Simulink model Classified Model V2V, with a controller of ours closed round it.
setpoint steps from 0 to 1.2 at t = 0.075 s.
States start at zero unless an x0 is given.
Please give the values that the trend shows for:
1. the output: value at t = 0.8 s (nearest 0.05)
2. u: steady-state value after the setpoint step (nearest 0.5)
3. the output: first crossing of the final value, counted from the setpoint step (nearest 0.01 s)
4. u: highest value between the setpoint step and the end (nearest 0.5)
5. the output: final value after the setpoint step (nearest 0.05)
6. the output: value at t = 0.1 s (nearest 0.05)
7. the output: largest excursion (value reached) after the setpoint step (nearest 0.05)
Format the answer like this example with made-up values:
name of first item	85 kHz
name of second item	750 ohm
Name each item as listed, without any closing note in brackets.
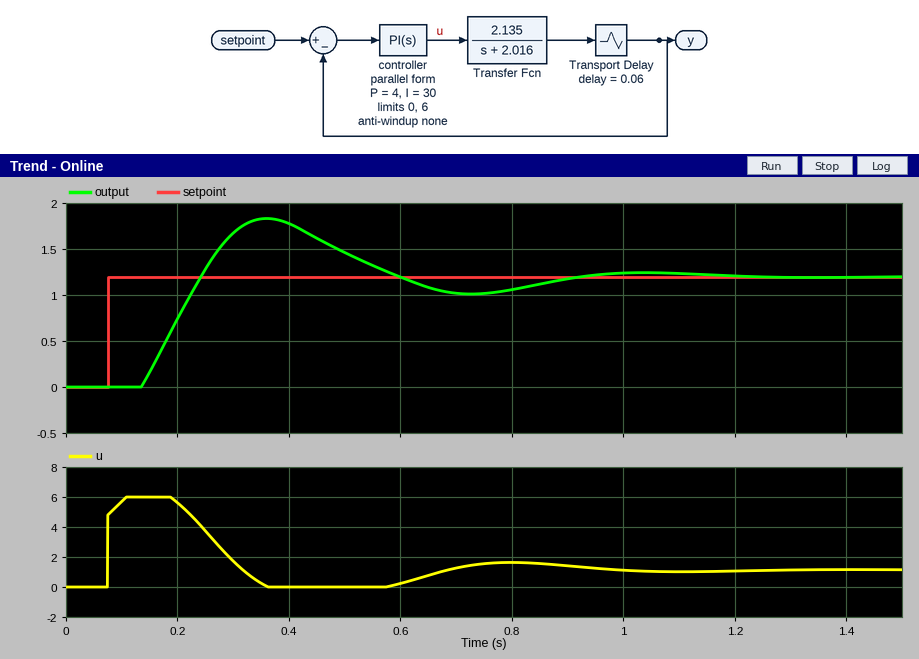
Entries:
the output: value at t = 0.8 s	1.05
u: steady-state value after the setpoint step	1.0
the output: first crossing of the final value, counted from the setpoint step	0.17 s
u: highest value between the setpoint step and the end	6.0
the output: final value after the setpoint step	1.20
the output: value at t = 0.1 s	0.00
the output: largest excursion (value reached) after the setpoint step	1.85
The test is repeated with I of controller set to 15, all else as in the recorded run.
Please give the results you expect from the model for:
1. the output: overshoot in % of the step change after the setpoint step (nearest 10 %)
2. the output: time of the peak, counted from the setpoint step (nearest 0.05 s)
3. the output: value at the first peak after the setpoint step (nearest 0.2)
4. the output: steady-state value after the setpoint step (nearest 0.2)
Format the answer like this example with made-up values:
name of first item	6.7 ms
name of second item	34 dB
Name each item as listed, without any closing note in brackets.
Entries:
the output: overshoot in % of the step change after the setpoint step	20 %
the output: time of the peak, counted from the setpoint step	0.30 s
the output: value at the first peak after the setpoint step	1.4
the output: steady-state value after the setpoint step	1.2
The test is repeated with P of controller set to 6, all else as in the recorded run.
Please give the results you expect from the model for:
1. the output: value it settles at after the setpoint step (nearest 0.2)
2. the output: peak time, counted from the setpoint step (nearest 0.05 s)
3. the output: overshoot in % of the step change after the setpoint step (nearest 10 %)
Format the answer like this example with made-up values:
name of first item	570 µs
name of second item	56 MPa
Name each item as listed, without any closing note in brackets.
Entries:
the output: value it settles at after the setpoint step	1.2
the output: peak time, counted from the setpoint step	0.25 s
the output: overshoot in % of the step change after the setpoint step	50 %
